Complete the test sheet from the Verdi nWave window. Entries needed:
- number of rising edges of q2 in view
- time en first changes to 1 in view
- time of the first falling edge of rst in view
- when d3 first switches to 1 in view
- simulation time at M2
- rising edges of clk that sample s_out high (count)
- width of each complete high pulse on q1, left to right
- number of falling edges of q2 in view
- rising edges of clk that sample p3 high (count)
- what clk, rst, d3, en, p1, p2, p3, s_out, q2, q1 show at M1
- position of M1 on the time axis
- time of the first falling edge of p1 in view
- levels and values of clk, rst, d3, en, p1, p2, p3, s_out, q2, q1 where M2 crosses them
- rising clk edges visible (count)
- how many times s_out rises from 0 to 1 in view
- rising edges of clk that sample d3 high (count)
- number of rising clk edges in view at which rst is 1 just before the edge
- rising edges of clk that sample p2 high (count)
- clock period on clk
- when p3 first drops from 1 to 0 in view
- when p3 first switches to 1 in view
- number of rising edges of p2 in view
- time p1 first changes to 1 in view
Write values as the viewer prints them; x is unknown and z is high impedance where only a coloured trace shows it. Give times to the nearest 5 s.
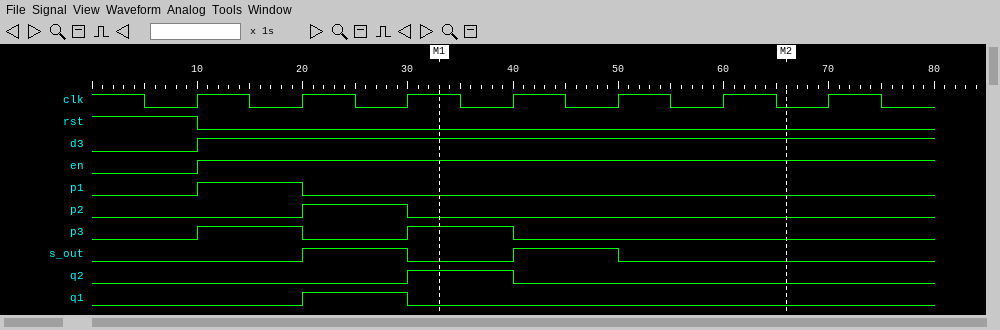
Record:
1
10 s
10 s
10 s
65 s
2
10 s
1
2
clk=1, rst=0, d3=1, en=1, p1=0, p2=0, p3=1, s_out=0, q2=1, q1=0
35 s
20 s
clk=0, rst=0, d3=1, en=1, p1=0, p2=0, p3=0, s_out=0, q2=0, q1=0
7
2
6
1
1
10 s
20 s
10 s
1
10 s
